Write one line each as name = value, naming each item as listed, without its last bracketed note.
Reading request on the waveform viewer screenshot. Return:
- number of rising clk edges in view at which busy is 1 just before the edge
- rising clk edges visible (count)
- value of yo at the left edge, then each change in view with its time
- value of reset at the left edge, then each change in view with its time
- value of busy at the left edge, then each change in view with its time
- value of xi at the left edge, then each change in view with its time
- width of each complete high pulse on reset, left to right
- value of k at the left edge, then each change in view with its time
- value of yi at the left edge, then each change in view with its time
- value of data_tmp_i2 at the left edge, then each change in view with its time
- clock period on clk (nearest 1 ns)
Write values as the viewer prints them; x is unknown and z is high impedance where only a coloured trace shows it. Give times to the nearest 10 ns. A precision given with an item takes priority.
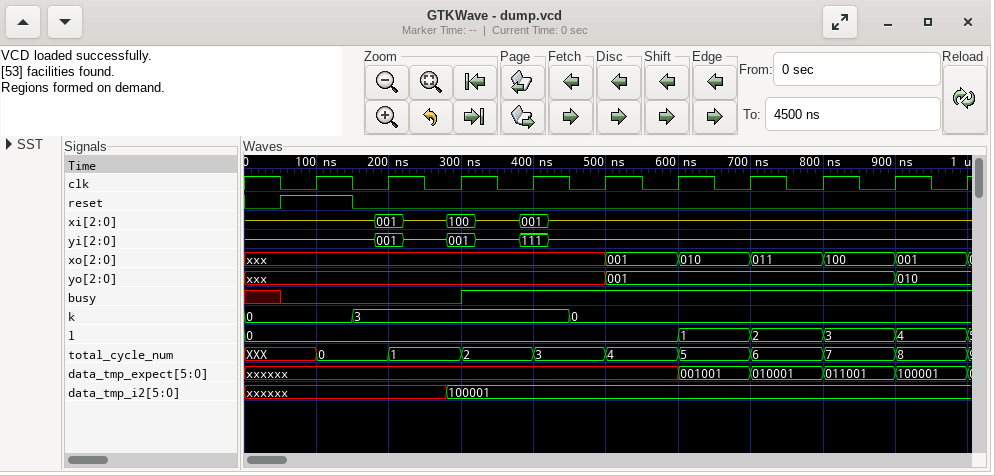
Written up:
number of rising clk edges in view at which busy is 1 just before the edge = 7
rising clk edges visible = 10
value of yo at the left edge, then each change in view with its time = xxx, 001 at 500 ns, 010 at 900 ns
value of reset at the left edge, then each change in view with its time = 0, 1 at 50 ns, 0 at 150 ns
value of busy at the left edge, then each change in view with its time = x, 0 at 50 ns, 1 at 300 ns
value of xi at the left edge, then each change in view with its time = z, 001 at 180 ns, z at 220 ns, 100 at 280 ns, z at 320 ns, 001 at 380 ns, z at 420 ns
width of each complete high pulse on reset, left to right = 100 ns
value of k at the left edge, then each change in view with its time = 0, 3 at 150 ns, 0 at 450 ns
value of yi at the left edge, then each change in view with its time = z, 001 at 180 ns, z at 220 ns, 001 at 280 ns, z at 320 ns, 111 at 380 ns, z at 420 ns
value of data_tmp_i2 at the left edge, then each change in view with its time = xxxxxx, 100001 at 280 ns
clock period on clk = 100 ns
